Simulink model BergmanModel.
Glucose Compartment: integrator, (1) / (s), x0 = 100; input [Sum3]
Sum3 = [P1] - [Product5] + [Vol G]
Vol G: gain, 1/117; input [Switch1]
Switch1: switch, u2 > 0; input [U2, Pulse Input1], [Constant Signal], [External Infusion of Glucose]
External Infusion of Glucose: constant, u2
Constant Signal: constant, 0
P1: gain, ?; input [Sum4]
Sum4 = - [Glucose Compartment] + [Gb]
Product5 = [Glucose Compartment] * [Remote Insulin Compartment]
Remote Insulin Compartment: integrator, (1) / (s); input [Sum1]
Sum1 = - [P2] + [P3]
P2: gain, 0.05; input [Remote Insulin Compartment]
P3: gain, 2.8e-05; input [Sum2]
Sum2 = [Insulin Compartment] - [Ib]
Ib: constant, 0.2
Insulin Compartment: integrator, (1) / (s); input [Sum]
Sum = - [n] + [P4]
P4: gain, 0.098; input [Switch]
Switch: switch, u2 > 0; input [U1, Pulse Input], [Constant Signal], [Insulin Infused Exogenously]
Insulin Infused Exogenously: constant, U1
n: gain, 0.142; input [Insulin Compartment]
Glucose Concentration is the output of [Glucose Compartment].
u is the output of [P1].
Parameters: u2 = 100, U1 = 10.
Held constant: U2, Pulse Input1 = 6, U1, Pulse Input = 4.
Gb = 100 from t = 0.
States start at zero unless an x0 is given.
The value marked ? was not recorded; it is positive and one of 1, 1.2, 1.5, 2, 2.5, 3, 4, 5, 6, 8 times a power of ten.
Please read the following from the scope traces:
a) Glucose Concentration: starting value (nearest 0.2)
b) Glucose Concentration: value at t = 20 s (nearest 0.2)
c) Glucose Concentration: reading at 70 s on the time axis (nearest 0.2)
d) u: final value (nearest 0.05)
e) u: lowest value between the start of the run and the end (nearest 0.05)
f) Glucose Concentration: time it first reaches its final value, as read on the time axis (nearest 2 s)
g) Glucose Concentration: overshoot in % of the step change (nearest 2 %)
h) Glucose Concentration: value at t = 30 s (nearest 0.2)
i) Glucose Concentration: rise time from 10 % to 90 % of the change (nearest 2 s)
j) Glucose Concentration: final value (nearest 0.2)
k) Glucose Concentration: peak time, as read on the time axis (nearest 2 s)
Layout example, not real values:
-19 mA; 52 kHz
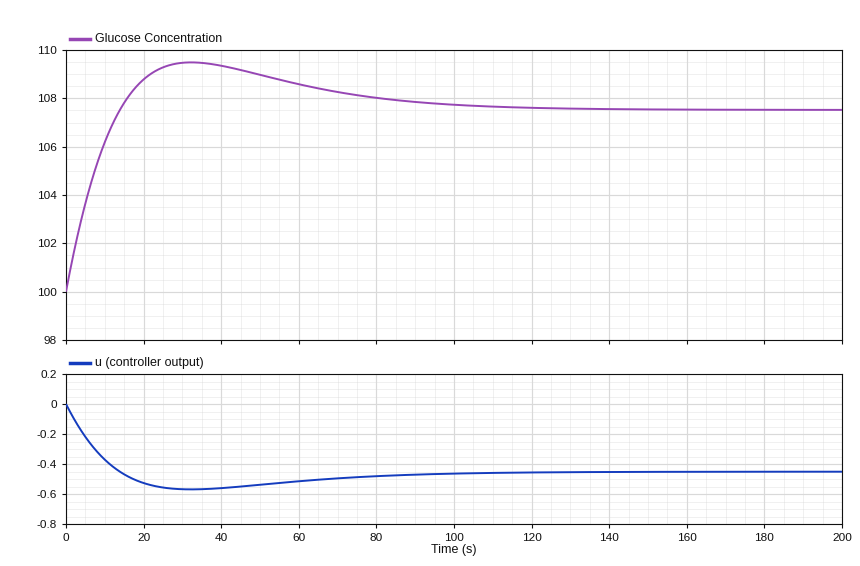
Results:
100.0; 108.8; 108.2; -0.45; -0.55; 14 s; 26 %; 109.4; 10 s; 107.6; 32 s
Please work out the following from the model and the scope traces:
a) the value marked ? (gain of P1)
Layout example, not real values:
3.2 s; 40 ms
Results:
0.06
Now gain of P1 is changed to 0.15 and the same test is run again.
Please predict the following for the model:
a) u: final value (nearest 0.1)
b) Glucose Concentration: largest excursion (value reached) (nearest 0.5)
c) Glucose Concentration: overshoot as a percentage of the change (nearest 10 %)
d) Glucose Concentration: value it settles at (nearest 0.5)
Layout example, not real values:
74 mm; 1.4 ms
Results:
-0.5; 104.5; 50 %; 103.0
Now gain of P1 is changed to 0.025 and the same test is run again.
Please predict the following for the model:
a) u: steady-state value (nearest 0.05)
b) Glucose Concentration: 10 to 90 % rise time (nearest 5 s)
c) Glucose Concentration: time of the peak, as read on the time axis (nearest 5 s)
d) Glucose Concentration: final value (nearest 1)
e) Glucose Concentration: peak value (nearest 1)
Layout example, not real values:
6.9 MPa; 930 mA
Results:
-0.40; 30 s; 70 s; 117; 117
